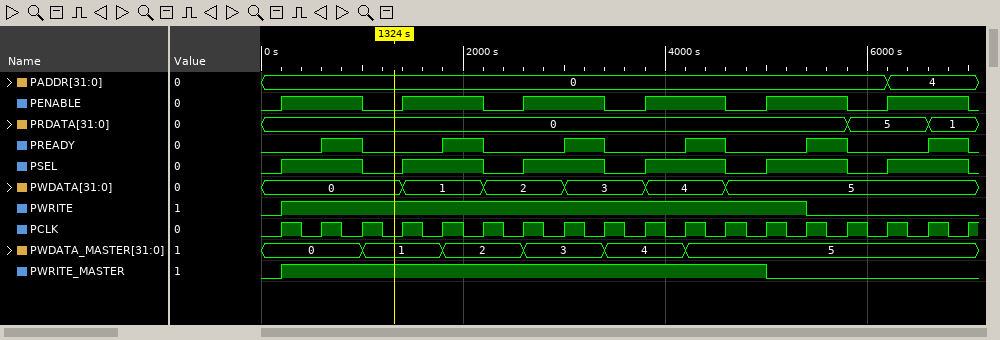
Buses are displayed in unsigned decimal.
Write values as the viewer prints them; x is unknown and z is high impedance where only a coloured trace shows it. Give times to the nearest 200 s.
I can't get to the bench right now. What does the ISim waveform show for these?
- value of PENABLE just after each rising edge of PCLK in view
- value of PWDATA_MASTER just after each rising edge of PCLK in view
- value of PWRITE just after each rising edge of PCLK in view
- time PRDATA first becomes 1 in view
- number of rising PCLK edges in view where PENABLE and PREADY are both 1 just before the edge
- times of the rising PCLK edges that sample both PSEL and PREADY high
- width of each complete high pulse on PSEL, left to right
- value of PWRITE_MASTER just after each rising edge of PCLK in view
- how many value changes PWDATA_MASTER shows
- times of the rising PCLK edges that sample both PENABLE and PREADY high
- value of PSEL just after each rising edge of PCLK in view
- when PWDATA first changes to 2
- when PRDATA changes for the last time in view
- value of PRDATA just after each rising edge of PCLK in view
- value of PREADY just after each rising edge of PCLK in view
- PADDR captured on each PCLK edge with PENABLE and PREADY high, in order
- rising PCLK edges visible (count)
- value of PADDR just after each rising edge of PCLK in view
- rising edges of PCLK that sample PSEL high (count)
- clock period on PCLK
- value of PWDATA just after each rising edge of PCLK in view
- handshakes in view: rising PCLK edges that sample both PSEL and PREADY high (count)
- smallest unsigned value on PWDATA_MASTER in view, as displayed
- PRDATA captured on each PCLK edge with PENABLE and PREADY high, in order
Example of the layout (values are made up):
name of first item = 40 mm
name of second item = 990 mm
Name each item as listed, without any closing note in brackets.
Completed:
value of PENABLE just after each rising edge of PCLK in view = 1 1 0 1 1 0 1 1 0 1 1 0 1 1 0 1 1 0
value of PWDATA_MASTER just after each rising edge of PCLK in view = 0, 0, 1, 1, 2, 2, 3, 3, 4, 4, 5, 5, 5, 5, 5, 5, 5, 5
value of PWRITE just after each rising edge of PCLK in view = 1 1 1 1 1 1 1 1 1 1 1 1 1 0 0 0 0 0
time PRDATA first becomes 1 in view = 6600 s
number of rising PCLK edges in view where PENABLE and PREADY are both 1 just before the edge = 6
times of the rising PCLK edges that sample both PSEL and PREADY high = 1000 s, 2200 s, 3400 s, 4600 s, 5800 s, 7000 s
width of each complete high pulse on PSEL, left to right = 800 s, 800 s, 800 s, 800 s, 800 s, 800 s
value of PWRITE_MASTER just after each rising edge of PCLK in view = 1 1 1 1 1 1 1 1 1 1 1 1 0 0 0 0 0 0
how many value changes PWDATA_MASTER shows = 5
times of the rising PCLK edges that sample both PENABLE and PREADY high = 1000 s, 2200 s, 3400 s, 4600 s, 5800 s, 7000 s
value of PSEL just after each rising edge of PCLK in view = 1 1 0 1 1 0 1 1 0 1 1 0 1 1 0 1 1 0
when PWDATA first changes to 2 = 2200 s
when PRDATA changes for the last time in view = 6600 s
value of PRDATA just after each rising edge of PCLK in view = 0, 0, 0, 0, 0, 0, 0, 0, 0, 0, 0, 0, 0, 0, 5, 5, 1, 1
value of PREADY just after each rising edge of PCLK in view = 0 1 0 0 1 0 0 1 0 0 1 0 0 1 0 0 1 0
PADDR captured on each PCLK edge with PENABLE and PREADY high, in order = 0, 0, 0, 0, 0, 4
rising PCLK edges visible = 18
value of PADDR just after each rising edge of PCLK in view = 0, 0, 0, 0, 0, 0, 0, 0, 0, 0, 0, 0, 0, 0, 0, 4, 4, 4
rising edges of PCLK that sample PSEL high = 12
clock period on PCLK = 400 s
value of PWDATA just after each rising edge of PCLK in view = 0, 0, 0, 1, 1, 2, 2, 3, 3, 4, 4, 5, 5, 5, 5, 5, 5, 5
handshakes in view: rising PCLK edges that sample both PSEL and PREADY high = 6
smallest unsigned value on PWDATA_MASTER in view, as displayed = 0
PRDATA captured on each PCLK edge with PENABLE and PREADY high, in order = 0, 0, 0, 0, 0, 1
